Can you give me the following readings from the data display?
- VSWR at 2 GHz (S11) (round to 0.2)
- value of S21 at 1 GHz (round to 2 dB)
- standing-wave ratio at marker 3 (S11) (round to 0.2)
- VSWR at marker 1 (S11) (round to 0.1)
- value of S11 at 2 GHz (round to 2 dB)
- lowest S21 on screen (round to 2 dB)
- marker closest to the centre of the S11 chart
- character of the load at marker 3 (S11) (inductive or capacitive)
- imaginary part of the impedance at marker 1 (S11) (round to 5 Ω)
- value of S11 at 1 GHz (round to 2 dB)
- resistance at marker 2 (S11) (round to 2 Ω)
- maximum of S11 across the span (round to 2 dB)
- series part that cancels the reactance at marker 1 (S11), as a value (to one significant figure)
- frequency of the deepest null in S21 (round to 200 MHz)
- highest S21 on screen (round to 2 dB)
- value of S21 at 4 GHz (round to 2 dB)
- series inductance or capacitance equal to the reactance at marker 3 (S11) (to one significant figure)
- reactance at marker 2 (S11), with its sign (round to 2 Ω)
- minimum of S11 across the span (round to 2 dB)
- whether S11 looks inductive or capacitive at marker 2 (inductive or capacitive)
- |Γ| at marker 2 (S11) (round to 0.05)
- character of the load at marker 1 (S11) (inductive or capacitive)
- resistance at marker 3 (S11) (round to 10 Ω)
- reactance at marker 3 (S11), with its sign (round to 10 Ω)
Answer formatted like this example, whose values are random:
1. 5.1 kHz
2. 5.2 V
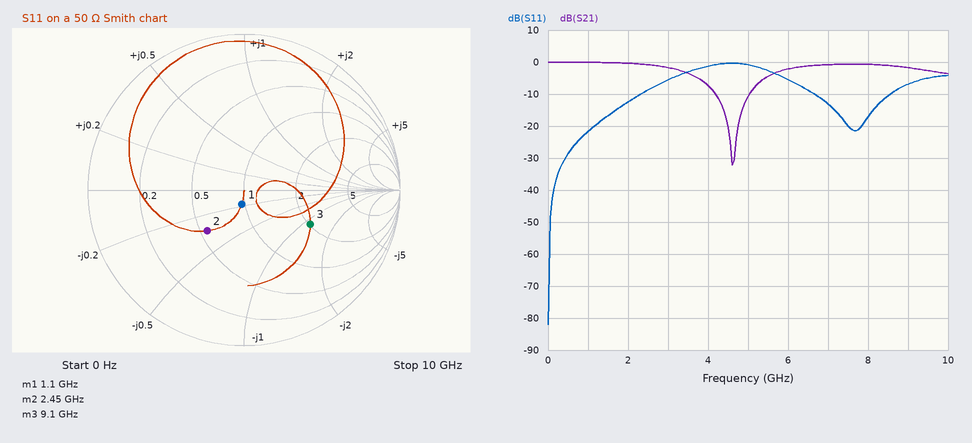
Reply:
1. 1.6
2. 0 dB
3. 2.8
4. 1.2
5. -12 dB
6. -32 dB
7. marker 1
8. capacitive
9. -10 Ω
10. -22 dB
11. 28 Ω
12. 0 dB
13. 1 nH
14. 4.6 GHz
15. 0 dB
16. -8 dB
17. 300 fF
18. -16 Ω
19. -82 dB
20. capacitive
21. 0.35
22. capacitive
23. 100 Ω
24. -60 Ω
